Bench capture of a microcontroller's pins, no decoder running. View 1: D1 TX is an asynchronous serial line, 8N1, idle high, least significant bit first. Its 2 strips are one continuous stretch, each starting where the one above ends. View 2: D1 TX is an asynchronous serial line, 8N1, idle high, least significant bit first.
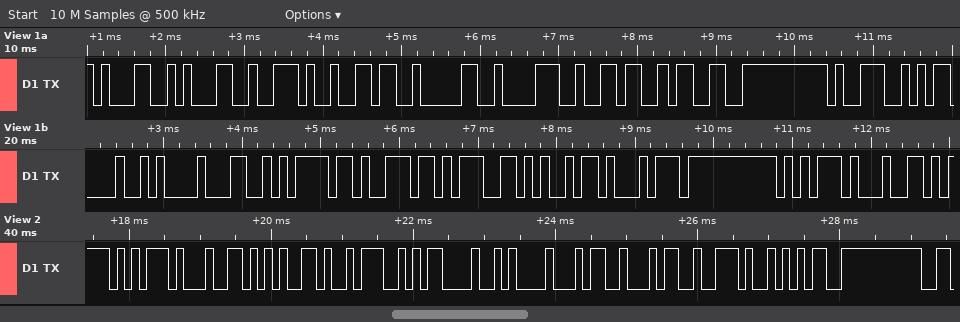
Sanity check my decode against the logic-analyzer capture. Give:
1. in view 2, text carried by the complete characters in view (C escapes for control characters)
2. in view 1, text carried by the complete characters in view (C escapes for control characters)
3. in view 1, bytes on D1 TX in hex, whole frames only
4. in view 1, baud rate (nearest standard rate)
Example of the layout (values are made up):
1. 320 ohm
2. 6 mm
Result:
1. "ude:\r\n44.5"
2. "11.608639\r\nLongitud"
3. 31 31 2E 36 30 38 36 33 39 0D 0A 4C 6F 6E 67 69 74 75 64
4. 9600 baud
